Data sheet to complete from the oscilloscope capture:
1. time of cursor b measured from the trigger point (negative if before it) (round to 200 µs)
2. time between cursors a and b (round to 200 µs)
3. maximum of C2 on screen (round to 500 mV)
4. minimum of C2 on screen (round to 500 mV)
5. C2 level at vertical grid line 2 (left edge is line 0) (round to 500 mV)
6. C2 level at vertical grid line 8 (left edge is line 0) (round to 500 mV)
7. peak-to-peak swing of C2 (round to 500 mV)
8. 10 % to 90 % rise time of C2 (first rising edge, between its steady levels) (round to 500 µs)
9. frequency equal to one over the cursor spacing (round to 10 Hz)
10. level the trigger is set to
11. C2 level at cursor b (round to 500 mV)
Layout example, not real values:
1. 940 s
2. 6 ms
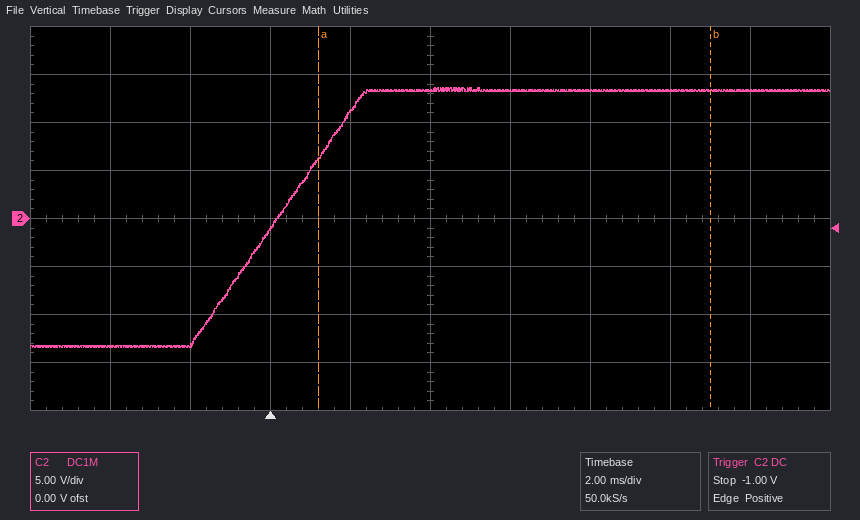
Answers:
1. +11.0 ms
2. 9.8 ms
3. 13.5 V
4. -13.5 V
5. -13.0 V
6. 13.5 V
7. 27.0 V
8. 3.5 ms
9. 100 Hz
10. -1.00 V
11. 13.5 V
